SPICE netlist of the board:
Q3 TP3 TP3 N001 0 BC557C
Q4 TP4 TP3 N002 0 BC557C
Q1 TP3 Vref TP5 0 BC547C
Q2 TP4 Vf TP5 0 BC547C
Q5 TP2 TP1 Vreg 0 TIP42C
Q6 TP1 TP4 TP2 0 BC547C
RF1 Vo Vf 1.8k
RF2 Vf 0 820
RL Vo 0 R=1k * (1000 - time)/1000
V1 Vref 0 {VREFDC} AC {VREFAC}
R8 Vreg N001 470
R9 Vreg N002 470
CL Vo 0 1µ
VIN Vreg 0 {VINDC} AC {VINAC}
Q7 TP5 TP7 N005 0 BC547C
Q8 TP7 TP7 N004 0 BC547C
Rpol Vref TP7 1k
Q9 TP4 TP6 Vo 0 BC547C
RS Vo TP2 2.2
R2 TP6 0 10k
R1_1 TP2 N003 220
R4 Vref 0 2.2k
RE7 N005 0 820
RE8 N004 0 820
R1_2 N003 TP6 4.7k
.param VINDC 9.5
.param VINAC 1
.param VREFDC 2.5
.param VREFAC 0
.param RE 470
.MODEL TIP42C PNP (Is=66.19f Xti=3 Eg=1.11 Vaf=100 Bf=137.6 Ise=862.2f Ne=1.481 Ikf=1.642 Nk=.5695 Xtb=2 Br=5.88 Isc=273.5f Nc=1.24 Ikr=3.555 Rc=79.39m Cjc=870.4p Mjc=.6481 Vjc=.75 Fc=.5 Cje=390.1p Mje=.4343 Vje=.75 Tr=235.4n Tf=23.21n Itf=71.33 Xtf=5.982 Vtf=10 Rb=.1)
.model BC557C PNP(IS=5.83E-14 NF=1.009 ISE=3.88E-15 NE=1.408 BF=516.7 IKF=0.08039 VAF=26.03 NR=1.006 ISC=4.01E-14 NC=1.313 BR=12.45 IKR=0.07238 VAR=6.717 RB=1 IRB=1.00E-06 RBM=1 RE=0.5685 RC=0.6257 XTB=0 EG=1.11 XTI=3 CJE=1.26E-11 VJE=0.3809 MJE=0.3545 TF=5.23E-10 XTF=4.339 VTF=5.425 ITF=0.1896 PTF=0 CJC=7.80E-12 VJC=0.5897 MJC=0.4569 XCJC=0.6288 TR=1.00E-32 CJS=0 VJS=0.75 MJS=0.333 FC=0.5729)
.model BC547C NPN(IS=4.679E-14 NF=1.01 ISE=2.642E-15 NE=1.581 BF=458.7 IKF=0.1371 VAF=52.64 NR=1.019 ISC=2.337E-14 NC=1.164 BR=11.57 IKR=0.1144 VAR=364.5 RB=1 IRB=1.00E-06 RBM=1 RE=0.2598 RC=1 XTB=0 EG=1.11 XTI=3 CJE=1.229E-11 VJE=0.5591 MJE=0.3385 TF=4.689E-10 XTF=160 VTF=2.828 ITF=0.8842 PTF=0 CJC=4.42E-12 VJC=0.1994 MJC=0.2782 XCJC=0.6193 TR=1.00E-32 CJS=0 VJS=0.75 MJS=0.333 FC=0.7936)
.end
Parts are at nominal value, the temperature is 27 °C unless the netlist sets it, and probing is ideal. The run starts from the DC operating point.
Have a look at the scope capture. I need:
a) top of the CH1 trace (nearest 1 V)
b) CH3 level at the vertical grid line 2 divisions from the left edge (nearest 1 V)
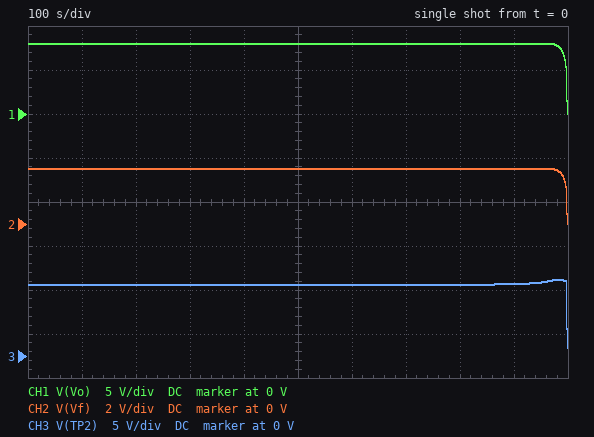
8 V
8 V
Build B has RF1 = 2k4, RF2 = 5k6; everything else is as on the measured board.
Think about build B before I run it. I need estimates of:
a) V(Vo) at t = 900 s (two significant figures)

3.6 V
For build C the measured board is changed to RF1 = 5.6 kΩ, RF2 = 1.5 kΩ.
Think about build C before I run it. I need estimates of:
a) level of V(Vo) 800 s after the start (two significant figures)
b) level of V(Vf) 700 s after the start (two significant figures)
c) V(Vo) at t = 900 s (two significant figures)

8.6 V
1.8 V
8.5 V
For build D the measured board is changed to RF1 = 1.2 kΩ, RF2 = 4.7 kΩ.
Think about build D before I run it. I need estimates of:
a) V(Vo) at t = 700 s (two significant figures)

3.1 V
